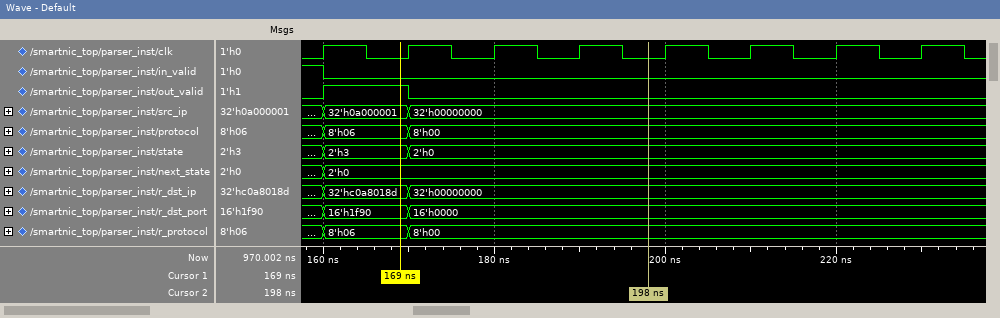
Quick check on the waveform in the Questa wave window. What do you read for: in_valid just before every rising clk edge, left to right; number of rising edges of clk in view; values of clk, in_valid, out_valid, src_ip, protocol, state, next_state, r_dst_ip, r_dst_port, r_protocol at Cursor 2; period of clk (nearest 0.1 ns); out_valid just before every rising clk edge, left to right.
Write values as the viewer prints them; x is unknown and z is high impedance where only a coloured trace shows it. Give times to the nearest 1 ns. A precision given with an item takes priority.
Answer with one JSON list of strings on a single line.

["1 0 0 0 0 0 0 0", "8", "clk=0, in_valid=0, out_valid=0, src_ip=32'h00000000, protocol=8'h00, state=2'h0, next_state=2'h0, r_dst_ip=32'h00000000, r_dst_port=16'h0000, r_protocol=8'h00", "10 ns", "0 1 0 0 0 0 0 0"]
